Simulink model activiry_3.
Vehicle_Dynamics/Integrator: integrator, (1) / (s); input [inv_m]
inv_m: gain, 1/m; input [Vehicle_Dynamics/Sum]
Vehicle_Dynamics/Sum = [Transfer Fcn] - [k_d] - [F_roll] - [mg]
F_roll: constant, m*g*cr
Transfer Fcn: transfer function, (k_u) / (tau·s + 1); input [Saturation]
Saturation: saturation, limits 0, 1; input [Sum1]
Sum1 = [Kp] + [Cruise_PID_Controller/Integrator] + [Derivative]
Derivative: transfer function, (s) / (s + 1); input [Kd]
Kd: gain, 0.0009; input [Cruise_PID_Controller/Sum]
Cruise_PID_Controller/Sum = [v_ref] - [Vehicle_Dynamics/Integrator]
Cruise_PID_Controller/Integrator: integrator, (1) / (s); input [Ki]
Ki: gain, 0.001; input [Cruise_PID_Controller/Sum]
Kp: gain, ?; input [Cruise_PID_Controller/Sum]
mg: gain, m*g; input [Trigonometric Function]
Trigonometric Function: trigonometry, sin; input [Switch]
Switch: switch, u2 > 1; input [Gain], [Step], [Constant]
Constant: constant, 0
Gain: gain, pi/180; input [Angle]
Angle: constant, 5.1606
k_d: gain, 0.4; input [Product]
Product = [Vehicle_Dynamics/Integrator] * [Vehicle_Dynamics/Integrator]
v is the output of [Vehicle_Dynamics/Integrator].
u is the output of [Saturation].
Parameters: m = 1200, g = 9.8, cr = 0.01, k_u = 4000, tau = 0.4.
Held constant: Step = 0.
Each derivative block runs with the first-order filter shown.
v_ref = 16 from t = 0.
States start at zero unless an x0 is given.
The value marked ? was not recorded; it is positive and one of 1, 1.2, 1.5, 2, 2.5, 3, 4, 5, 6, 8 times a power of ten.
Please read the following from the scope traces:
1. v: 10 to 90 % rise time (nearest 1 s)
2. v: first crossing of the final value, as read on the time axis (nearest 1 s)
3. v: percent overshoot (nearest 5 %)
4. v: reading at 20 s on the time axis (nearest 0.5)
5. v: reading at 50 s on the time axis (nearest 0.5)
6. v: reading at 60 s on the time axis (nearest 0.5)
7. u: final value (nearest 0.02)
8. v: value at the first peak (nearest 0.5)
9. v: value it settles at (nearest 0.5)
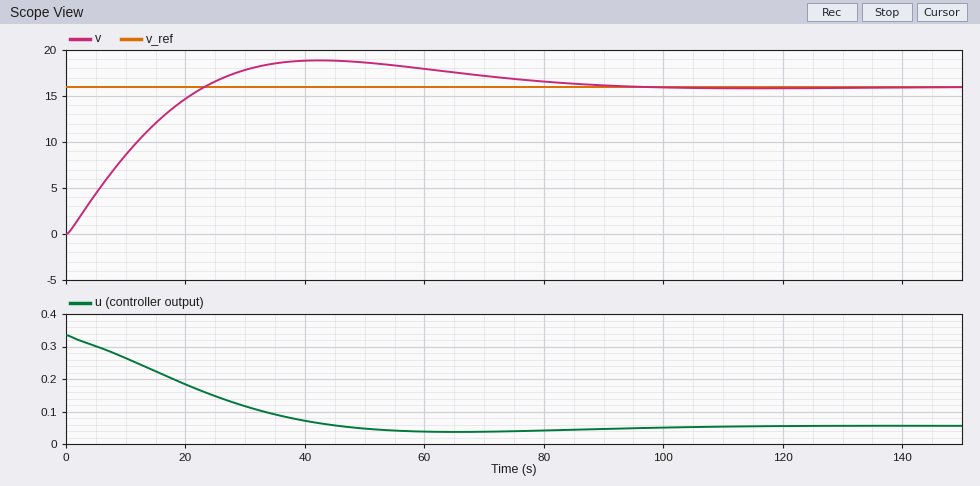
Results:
17 s
23 s
20 %
14.5
18.5
18.0
0.06
19.0
16.0
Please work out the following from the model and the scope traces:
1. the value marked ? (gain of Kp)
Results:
0.02
